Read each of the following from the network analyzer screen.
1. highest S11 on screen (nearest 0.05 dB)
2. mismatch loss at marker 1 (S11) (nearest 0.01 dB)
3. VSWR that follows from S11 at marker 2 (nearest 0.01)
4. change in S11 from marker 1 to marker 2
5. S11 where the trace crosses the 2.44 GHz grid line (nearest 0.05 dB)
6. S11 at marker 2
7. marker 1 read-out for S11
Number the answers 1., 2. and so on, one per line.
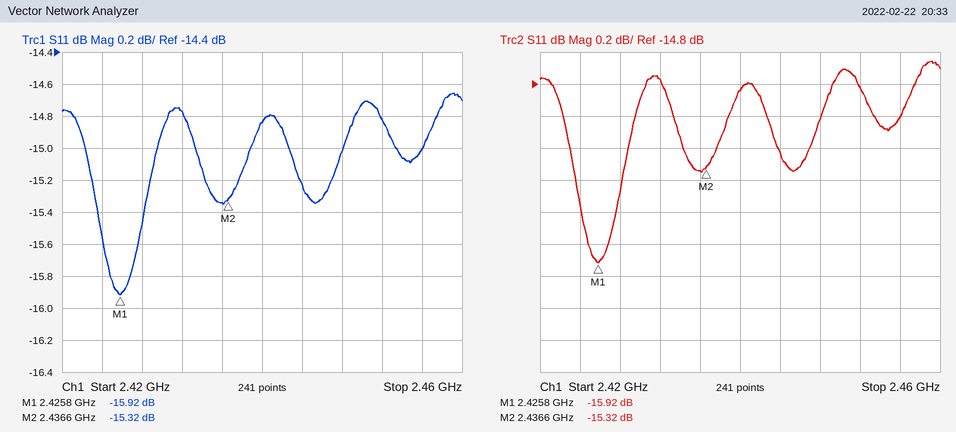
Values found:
1. -14.65 dB
2. 0.11 dB
3. 1.41
4. 0.60 dB
5. -14.85 dB
6. -15.32 dB
7. -15.92 dB
